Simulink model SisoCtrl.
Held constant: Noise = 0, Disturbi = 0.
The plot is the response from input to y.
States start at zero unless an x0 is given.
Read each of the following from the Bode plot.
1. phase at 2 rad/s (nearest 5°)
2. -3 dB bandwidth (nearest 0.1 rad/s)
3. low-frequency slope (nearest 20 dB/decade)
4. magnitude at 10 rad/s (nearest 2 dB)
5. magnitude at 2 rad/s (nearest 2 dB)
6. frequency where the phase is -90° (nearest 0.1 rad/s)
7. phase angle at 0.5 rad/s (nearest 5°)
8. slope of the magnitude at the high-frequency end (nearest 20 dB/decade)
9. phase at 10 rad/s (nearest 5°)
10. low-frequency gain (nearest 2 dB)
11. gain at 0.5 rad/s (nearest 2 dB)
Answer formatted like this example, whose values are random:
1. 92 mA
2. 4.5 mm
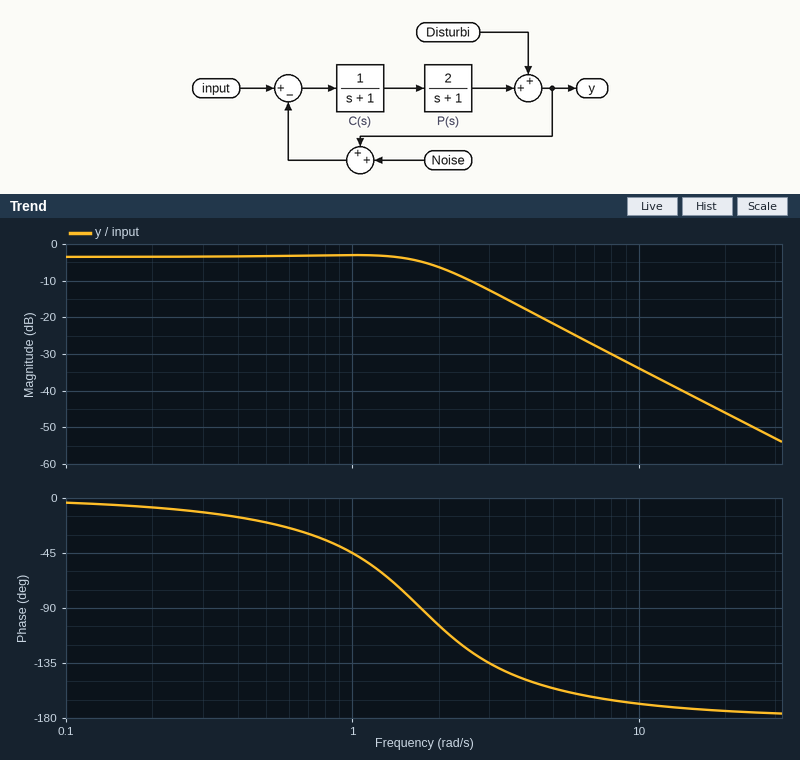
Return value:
1. -105°
2. 2.0 rad/s
3. 0 dB/decade
4. -34 dB
5. -6 dB
6. 1.7 rad/s
7. -20°
8. -40 dB/decade
9. -170°
10. -4 dB
11. -4 dB
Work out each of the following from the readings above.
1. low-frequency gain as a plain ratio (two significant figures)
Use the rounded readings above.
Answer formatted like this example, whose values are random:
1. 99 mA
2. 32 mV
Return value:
1. 0.63
